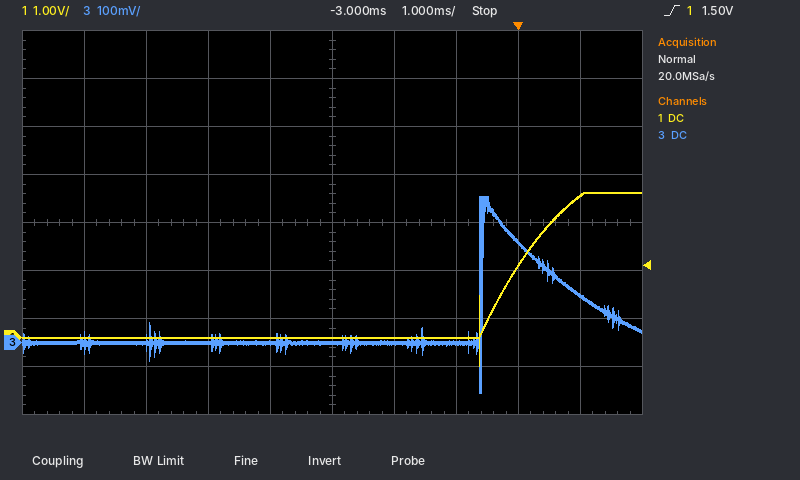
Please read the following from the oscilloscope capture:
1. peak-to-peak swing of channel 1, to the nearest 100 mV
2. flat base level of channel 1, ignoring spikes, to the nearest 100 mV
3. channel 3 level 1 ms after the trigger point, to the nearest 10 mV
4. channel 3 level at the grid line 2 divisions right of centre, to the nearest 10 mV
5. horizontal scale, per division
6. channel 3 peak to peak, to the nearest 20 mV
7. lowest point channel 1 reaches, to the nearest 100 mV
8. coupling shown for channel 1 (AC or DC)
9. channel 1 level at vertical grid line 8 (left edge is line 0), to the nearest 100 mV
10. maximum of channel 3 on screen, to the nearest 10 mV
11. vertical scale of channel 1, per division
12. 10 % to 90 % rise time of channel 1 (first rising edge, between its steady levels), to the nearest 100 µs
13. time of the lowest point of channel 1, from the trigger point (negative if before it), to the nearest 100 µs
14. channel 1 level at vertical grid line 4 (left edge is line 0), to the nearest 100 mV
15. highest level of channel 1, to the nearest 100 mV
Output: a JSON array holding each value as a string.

["3.6 V", "0.0 V", "100 mV", "0 mV", "1 ms", "400 mV", "-600 mV", "DC", "1.5 V", "300 mV", "1 V", "1.3 ms", "-600 µs", "0.0 V", "3.0 V"]
